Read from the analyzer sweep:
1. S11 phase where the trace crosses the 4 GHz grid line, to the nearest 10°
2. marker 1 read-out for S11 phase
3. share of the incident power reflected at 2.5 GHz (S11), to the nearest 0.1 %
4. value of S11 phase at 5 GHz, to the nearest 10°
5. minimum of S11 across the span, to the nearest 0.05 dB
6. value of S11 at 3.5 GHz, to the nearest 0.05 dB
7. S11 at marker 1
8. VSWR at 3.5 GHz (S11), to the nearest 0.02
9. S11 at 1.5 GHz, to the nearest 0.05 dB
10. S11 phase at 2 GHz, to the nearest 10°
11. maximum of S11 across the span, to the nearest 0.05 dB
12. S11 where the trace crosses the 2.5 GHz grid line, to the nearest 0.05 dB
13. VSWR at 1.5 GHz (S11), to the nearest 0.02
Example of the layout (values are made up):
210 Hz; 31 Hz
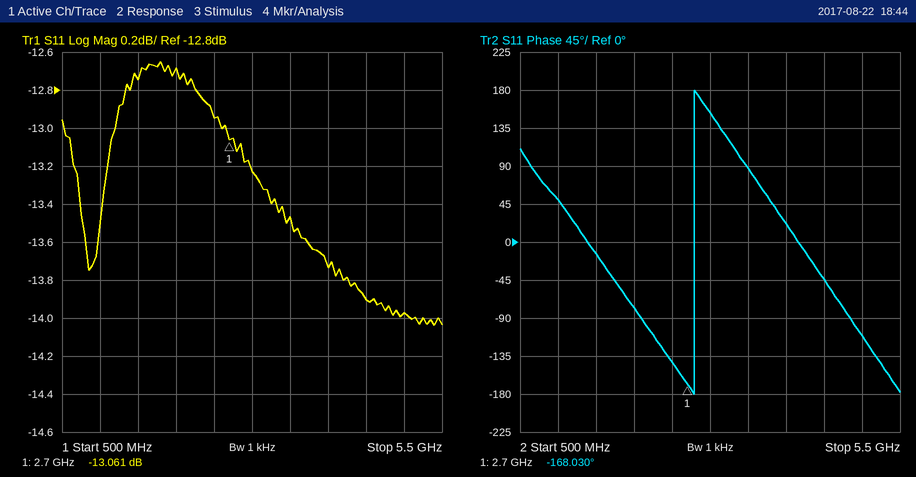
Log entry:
20°; -168.030°; 5.1 %; -110°; -14.05 dB; -13.45 dB; -13.061 dB; 1.54; -12.75 dB; -80°; -12.65 dB; -12.95 dB; 1.60
